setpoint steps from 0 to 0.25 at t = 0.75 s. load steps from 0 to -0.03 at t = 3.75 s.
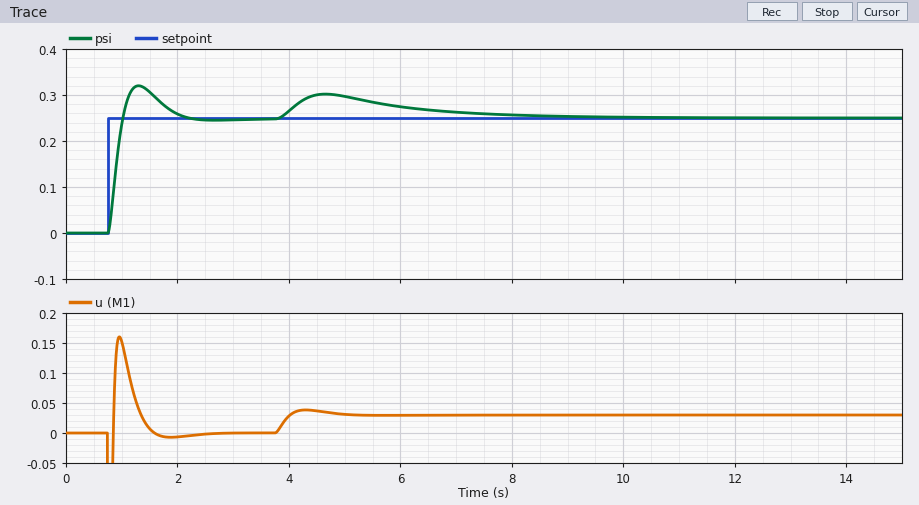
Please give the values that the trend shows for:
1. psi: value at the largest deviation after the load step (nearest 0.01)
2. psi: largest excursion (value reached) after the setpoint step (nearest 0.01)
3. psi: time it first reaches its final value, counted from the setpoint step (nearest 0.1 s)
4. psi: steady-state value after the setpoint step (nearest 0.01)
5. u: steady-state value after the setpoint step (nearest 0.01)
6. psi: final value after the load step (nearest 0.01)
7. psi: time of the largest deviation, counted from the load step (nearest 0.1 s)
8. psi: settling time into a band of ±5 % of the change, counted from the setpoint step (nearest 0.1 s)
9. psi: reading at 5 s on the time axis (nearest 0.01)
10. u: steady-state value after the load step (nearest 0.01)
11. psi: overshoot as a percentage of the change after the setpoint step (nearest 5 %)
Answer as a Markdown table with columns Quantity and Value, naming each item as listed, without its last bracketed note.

| Quantity | Value |
|---|---|
| psi: value at the largest deviation after the load step | 0.30 |
| psi: largest excursion (value reached) after the setpoint step | 0.32 |
| psi: time it first reaches its final value, counted from the setpoint step | 0.3 s |
| psi: steady-state value after the setpoint step | 0.25 |
| u: steady-state value after the setpoint step | 0.00 |
| psi: final value after the load step | 0.25 |
| psi: time of the largest deviation, counted from the load step | 0.9 s |
| psi: settling time into a band of ±5 % of the change, counted from the setpoint step | 1.2 s |
| psi: reading at 5 s on the time axis | 0.30 |
| u: steady-state value after the load step | 0.03 |
| psi: overshoot as a percentage of the change after the setpoint step | 30 % |
